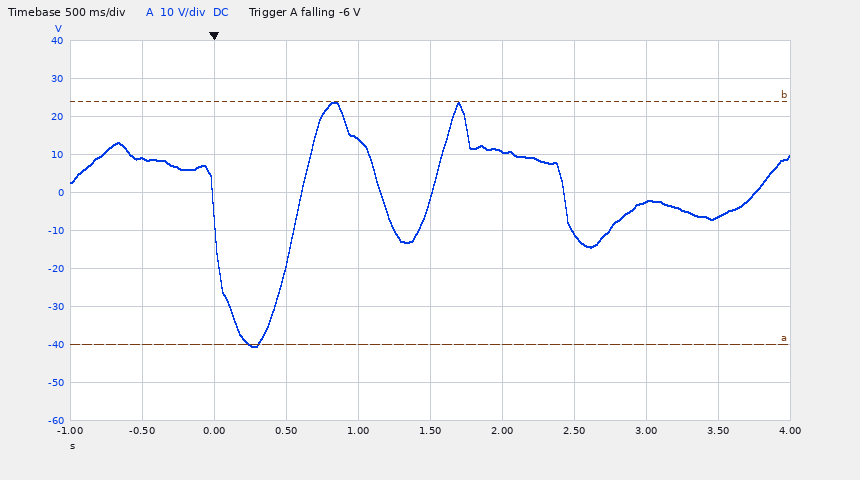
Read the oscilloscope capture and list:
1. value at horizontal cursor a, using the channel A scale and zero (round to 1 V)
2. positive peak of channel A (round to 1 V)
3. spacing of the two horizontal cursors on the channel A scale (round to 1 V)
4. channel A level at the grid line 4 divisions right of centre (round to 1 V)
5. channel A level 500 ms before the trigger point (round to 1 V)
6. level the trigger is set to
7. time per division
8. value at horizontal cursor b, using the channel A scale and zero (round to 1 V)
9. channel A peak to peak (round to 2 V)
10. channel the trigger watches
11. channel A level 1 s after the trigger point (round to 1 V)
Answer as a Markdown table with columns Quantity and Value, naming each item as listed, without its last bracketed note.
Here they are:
| Quantity | Value |
|---|---|
| value at horizontal cursor a, using the channel A scale and zero | -40 V |
| positive peak of channel A | 24 V |
| spacing of the two horizontal cursors on the channel A scale | 64 V |
| channel A level at the grid line 4 divisions right of centre | -6 V |
| channel A level 500 ms before the trigger point | 9 V |
| level the trigger is set to | -6 V |
| time per division | 500 ms |
| value at horizontal cursor b, using the channel A scale and zero | 24 V |
| channel A peak to peak | 64 V |
| channel the trigger watches | channel A |
| channel A level 1 s after the trigger point | 14 V |
